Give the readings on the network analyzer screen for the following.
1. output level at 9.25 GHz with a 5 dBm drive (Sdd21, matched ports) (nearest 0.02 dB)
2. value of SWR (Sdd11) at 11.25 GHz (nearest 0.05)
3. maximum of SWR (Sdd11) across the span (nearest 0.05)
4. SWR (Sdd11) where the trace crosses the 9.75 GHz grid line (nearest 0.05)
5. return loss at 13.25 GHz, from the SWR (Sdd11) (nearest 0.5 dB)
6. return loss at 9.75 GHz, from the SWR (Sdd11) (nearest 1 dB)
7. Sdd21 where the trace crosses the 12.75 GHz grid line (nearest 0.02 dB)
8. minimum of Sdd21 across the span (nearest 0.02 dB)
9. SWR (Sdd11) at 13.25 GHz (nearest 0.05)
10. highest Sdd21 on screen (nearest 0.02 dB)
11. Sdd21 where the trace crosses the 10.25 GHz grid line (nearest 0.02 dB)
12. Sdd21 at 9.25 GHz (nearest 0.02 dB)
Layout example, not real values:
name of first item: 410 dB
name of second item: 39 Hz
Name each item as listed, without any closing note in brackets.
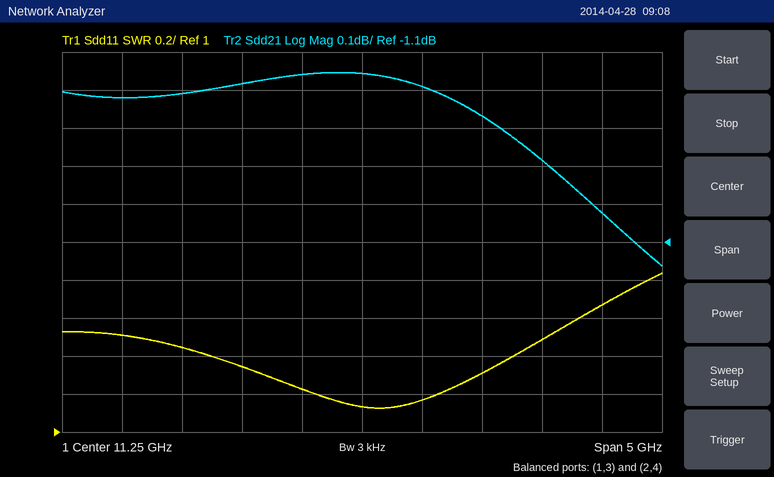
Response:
output level at 9.25 GHz with a 5 dBm drive (Sdd21, matched ports): 4.28 dBm
value of SWR (Sdd11) at 11.25 GHz: 1.15
maximum of SWR (Sdd11) across the span: 1.85
SWR (Sdd11) where the trace crosses the 9.75 GHz grid line: 1.45
return loss at 13.25 GHz, from the SWR (Sdd11): 12.0 dB
return loss at 9.75 GHz, from the SWR (Sdd11): 15 dB
Sdd21 where the trace crosses the 12.75 GHz grid line: -0.88 dB
minimum of Sdd21 across the span: -1.16 dB
SWR (Sdd11) at 13.25 GHz: 1.65
highest Sdd21 on screen: -0.66 dB
Sdd21 where the trace crosses the 10.25 GHz grid line: -0.68 dB
Sdd21 at 9.25 GHz: -0.72 dB
